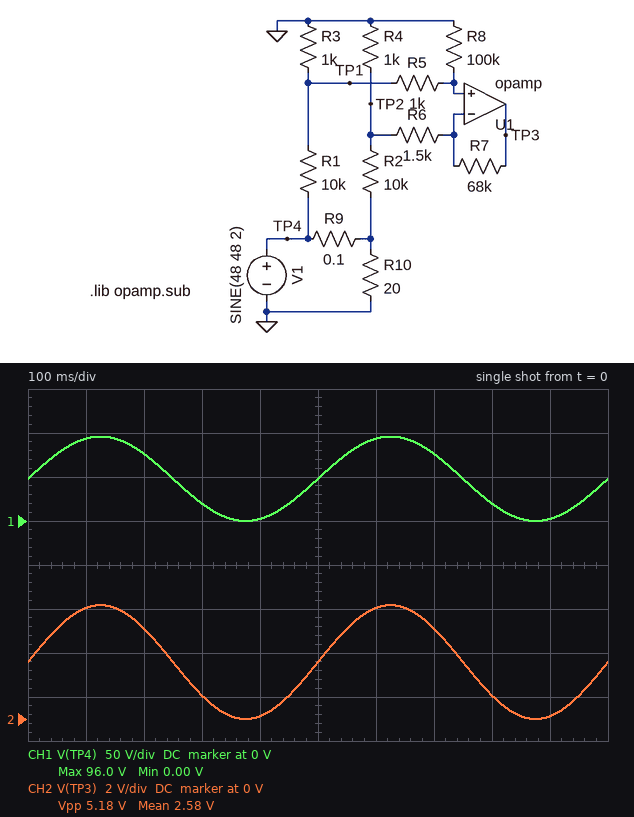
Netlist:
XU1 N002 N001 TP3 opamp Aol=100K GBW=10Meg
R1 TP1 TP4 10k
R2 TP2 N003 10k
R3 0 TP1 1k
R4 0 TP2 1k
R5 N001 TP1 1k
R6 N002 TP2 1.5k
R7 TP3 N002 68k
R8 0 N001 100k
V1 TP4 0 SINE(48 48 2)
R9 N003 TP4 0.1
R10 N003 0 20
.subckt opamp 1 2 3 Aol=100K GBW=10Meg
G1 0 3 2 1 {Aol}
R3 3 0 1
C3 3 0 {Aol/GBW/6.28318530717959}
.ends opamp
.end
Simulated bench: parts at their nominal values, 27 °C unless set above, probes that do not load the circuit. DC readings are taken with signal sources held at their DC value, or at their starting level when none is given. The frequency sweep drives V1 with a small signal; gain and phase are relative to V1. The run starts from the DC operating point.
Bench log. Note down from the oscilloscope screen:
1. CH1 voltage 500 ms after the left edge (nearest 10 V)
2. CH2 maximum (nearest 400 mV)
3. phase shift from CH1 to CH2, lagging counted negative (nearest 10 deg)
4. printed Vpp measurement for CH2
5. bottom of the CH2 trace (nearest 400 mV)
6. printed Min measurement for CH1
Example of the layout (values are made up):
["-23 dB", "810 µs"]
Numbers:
["50 V", "5.2 V", "0 deg", "5.18 V", "0 V", "0.00 V"]
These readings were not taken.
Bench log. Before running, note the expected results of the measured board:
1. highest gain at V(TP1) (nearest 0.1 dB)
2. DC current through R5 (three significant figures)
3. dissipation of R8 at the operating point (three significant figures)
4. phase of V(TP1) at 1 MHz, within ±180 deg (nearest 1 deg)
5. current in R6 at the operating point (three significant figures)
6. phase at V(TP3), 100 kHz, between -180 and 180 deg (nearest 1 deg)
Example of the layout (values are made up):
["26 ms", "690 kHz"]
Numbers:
["-20.9 dB", "42.8 µA", "183 µW", "0 deg", "24.9 µA", "-16 deg"]
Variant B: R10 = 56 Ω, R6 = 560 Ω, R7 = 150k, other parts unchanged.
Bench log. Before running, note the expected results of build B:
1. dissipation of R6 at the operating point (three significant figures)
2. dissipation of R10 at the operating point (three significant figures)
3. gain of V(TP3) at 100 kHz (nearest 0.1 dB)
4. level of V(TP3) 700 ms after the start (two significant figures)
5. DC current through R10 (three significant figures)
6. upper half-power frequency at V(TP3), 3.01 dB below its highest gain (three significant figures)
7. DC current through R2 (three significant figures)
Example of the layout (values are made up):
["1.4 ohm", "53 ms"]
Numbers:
["1.42 µW", "41.0 W", "-26.5 dB", "-5.2 V", "856 mA", "97.1 kHz", "4.36 mA"]
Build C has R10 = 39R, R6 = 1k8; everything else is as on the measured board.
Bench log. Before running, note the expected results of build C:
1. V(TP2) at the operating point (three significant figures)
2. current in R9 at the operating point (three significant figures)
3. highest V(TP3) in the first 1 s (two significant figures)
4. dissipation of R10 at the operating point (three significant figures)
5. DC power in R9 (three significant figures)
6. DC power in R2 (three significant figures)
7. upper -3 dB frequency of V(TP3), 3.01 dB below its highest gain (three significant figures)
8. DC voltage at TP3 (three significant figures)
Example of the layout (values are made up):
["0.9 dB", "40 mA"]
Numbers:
["4.33 V", "1.23 A", "5.0 V", "58.8 W", "152 mW", "190 mW", "383 kHz", "2.51 V"]
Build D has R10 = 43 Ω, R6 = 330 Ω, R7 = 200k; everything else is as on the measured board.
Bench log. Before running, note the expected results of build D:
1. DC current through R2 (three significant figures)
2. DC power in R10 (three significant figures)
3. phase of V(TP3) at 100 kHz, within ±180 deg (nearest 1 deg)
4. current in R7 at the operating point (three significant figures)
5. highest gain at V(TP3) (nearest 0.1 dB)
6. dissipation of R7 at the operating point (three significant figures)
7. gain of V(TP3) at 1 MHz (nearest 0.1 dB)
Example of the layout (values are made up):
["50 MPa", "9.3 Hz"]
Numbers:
["4.36 mA", "53.3 W", "122 deg", "57.7 µA", "-16.4 dB", "666 µW", "-40.6 dB"]
